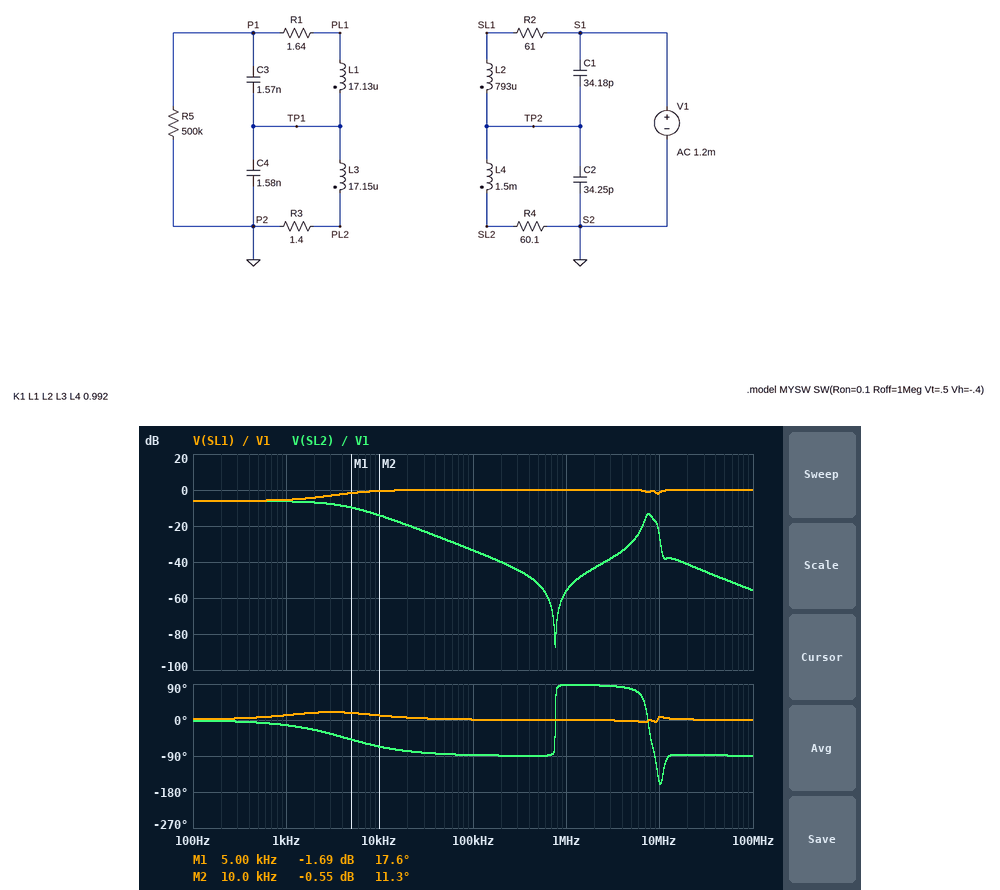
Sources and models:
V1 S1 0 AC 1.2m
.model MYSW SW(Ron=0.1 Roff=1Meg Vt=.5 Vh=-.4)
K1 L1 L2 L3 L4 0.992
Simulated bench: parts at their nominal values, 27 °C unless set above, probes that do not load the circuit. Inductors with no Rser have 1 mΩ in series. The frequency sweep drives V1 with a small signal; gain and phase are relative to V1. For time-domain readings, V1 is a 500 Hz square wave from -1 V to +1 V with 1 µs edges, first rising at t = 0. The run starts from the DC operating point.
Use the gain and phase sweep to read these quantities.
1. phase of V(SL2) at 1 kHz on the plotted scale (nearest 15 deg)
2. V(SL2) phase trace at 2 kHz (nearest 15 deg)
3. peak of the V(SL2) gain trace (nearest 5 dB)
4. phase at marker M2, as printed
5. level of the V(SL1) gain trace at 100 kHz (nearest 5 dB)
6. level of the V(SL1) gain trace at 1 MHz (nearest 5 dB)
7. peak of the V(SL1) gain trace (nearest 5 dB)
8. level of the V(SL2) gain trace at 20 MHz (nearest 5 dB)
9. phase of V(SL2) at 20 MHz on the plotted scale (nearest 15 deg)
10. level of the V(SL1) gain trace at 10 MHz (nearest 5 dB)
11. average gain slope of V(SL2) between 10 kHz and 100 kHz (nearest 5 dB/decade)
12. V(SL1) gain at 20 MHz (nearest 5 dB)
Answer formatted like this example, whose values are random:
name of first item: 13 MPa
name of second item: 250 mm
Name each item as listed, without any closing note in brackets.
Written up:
phase of V(SL2) at 1 kHz on the plotted scale: -15 deg
V(SL2) phase trace at 2 kHz: -30 deg
peak of the V(SL2) gain trace: -5 dB
phase at marker M2, as printed: 11.3 deg
level of the V(SL1) gain trace at 100 kHz: 0 dB
level of the V(SL1) gain trace at 1 MHz: 0 dB
peak of the V(SL1) gain trace: 0 dB
level of the V(SL2) gain trace at 20 MHz: -40 dB
phase of V(SL2) at 20 MHz on the plotted scale: -90 deg
level of the V(SL1) gain trace at 10 MHz: 0 dB
average gain slope of V(SL2) between 10 kHz and 100 kHz: -20 dB/decade
V(SL1) gain at 20 MHz: 0 dB
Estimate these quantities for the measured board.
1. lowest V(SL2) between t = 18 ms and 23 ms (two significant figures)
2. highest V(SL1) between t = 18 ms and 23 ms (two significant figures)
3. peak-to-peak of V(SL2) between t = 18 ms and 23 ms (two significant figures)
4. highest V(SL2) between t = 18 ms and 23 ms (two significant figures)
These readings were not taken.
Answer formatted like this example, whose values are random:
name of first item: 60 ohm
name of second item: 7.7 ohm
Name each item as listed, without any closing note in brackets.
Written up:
lowest V(SL2) between t = 18 ms and 23 ms: -500 mV
highest V(SL1) between t = 18 ms and 23 ms: 1.5 V
peak-to-peak of V(SL2) between t = 18 ms and 23 ms: 990 mV
highest V(SL2) between t = 18 ms and 23 ms: 500 mV
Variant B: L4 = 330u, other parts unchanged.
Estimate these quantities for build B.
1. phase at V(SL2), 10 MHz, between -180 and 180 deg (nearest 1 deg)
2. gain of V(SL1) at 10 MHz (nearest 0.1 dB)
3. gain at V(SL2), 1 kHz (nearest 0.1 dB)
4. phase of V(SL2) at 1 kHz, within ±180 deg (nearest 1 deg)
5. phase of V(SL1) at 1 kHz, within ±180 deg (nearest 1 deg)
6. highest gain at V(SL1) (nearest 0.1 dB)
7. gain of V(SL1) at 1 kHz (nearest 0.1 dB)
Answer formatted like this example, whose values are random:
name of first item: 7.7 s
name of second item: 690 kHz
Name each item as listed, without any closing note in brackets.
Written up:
phase at V(SL2), 10 MHz, between -180 and 180 deg: -40 deg
gain of V(SL1) at 10 MHz: -0.3 dB
gain at V(SL2), 1 kHz: -6.1 dB
phase of V(SL2) at 1 kHz, within ±180 deg: -6 deg
phase of V(SL1) at 1 kHz, within ±180 deg: 6 deg
highest gain at V(SL1): 0.8 dB
gain of V(SL1) at 1 kHz: -5.9 dB
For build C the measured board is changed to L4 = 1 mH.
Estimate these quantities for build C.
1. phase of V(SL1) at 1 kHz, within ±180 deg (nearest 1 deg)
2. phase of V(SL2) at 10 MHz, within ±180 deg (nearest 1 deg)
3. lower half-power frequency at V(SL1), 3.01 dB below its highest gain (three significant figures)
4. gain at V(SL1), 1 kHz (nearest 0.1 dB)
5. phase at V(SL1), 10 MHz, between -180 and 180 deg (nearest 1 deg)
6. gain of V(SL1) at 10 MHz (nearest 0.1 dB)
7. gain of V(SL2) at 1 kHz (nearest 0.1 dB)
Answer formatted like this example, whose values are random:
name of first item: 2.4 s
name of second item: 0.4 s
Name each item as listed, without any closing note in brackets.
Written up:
phase of V(SL1) at 1 kHz, within ±180 deg: 10 deg
phase of V(SL2) at 10 MHz, within ±180 deg: -99 deg
lower half-power frequency at V(SL1), 3.01 dB below its highest gain: 3.86 kHz
gain at V(SL1), 1 kHz: -5.7 dB
phase at V(SL1), 10 MHz, between -180 and 180 deg: 2 deg
gain of V(SL1) at 10 MHz: -0.7 dB
gain of V(SL2) at 1 kHz: -6.2 dB
